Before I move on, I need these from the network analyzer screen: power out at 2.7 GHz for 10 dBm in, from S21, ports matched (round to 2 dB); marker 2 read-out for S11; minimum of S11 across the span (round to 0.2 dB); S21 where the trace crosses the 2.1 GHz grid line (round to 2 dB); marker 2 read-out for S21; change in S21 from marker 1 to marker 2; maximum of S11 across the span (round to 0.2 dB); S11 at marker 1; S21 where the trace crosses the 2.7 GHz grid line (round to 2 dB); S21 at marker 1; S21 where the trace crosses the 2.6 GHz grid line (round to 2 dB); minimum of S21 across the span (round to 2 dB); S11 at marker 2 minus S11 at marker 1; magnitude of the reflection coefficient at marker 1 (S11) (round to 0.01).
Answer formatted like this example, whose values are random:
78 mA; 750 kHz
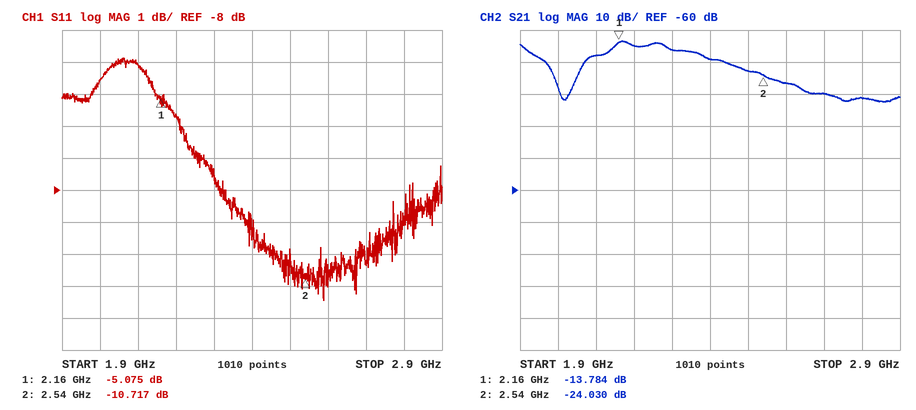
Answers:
-20 dBm; -10.717 dB; -11.4 dB; -18 dB; -24.030 dB; -10.246 dB; -3.8 dB; -5.075 dB; -30 dB; -13.784 dB; -26 dB; -32 dB; -5.642 dB; 0.56
